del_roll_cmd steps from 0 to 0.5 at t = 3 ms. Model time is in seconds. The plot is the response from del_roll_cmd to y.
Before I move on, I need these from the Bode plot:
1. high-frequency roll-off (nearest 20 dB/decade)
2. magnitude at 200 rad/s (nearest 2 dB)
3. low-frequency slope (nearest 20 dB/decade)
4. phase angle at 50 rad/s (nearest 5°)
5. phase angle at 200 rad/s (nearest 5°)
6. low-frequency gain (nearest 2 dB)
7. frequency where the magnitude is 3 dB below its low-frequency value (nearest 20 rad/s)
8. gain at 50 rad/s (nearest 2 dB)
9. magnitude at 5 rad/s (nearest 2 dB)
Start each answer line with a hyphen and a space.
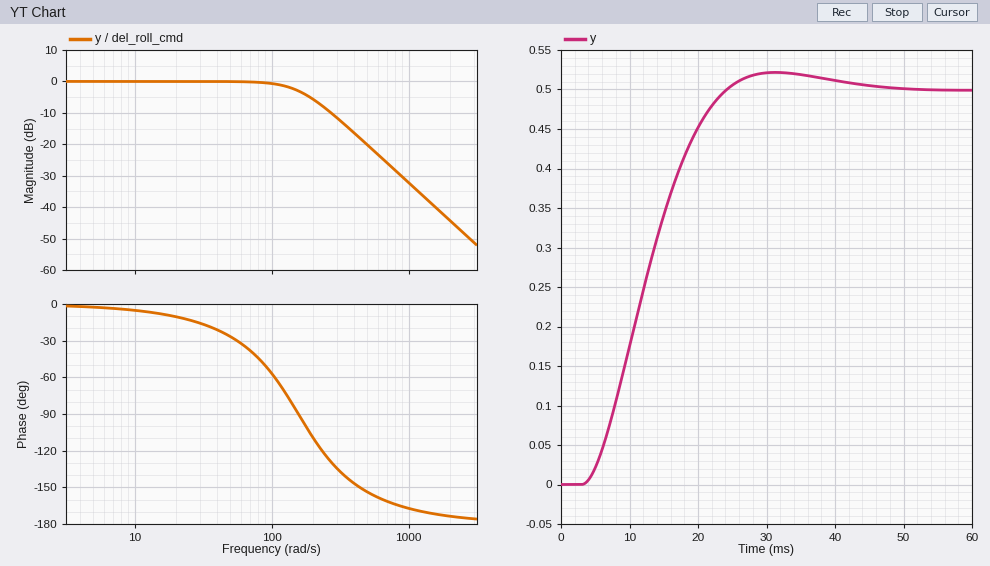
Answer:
- -40 dB/decade
- -6 dB
- 0 dB/decade
- -25°
- -110°
- 0 dB
- 160 rad/s
- 0 dB
- 0 dB
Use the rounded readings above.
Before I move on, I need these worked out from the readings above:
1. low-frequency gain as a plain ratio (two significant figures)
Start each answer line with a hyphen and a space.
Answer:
- 1.0
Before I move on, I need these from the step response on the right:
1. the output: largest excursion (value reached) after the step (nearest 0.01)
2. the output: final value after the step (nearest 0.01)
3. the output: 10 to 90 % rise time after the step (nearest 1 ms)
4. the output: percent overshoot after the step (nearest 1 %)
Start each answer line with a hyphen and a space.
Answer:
- 0.52
- 0.50
- 14 ms
- 4 %
